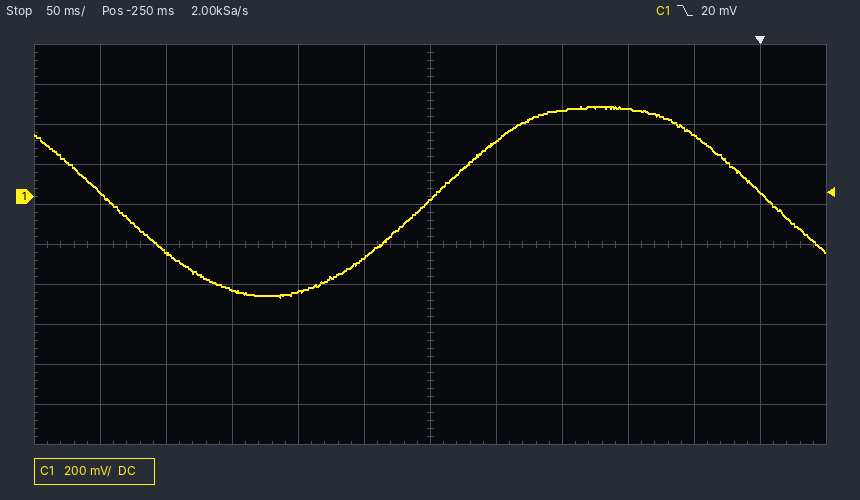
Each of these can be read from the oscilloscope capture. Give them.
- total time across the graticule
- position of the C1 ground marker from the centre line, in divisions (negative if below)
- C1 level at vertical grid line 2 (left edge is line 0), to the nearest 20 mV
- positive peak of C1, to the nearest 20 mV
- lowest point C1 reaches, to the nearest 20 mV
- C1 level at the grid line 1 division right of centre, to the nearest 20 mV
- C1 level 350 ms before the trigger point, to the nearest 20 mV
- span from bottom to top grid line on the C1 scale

600 ms
+1.2 div
-280 mV
440 mV
-500 mV
280 mV
-480 mV
2 V
